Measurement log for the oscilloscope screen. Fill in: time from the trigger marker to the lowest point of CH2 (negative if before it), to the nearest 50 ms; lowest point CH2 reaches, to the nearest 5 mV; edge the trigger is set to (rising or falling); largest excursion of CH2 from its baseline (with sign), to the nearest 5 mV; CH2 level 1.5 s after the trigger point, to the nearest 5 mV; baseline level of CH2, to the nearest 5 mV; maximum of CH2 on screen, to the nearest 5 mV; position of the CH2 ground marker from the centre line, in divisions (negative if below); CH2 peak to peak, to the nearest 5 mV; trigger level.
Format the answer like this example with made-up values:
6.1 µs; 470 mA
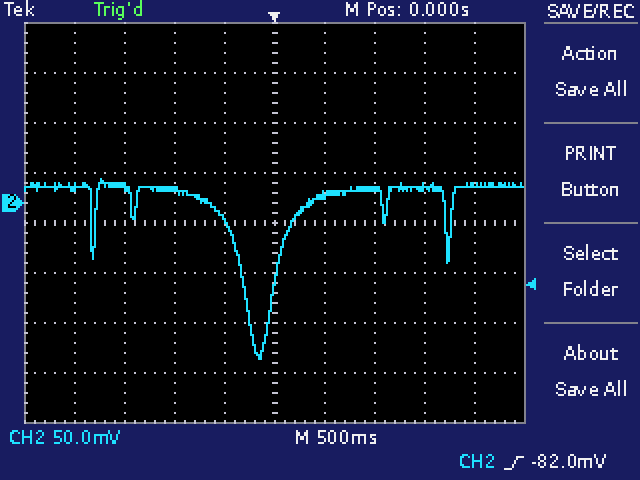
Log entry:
-150 ms; -155 mV; rising; -170 mV; 15 mV; 15 mV; 25 mV; +0.4 div; 180 mV; -82.0 mV
